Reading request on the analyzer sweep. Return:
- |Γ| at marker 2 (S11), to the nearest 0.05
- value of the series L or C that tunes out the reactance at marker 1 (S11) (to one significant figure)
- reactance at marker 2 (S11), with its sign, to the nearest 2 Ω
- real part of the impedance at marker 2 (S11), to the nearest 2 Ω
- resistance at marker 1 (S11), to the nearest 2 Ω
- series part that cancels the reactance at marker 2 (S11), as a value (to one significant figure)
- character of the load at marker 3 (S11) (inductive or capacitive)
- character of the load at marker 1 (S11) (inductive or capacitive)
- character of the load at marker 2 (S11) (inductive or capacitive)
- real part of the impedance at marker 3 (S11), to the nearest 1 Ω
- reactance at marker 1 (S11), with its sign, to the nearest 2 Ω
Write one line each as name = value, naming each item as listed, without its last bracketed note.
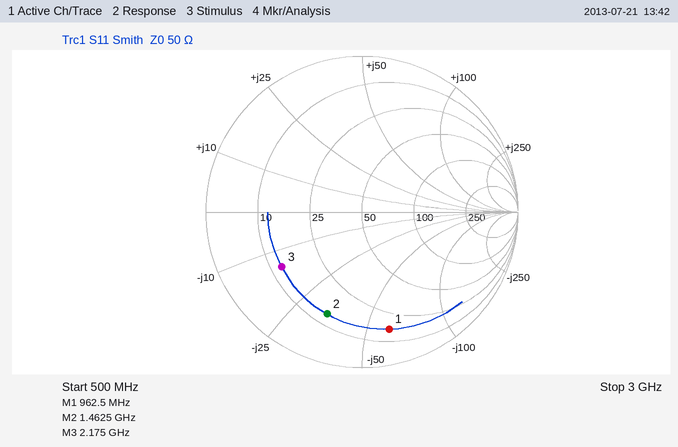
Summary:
|Γ| at marker 2 (S11), to the nearest 0.05 = 0.70
value of the series L or C that tunes out the reactance at marker 1 (S11) = 10 nH
reactance at marker 2 (S11), with its sign, to the nearest 2 Ω = -34 Ω
real part of the impedance at marker 2 (S11), to the nearest 2 Ω = 14 Ω
resistance at marker 1 (S11), to the nearest 2 Ω = 16 Ω
series part that cancels the reactance at marker 2 (S11), as a value = 4 nH
character of the load at marker 3 (S11) = capacitive
character of the load at marker 1 (S11) = capacitive
character of the load at marker 2 (S11) = capacitive
real part of the impedance at marker 3 (S11), to the nearest 1 Ω = 13 Ω
reactance at marker 1 (S11), with its sign, to the nearest 2 Ω = -60 Ω
